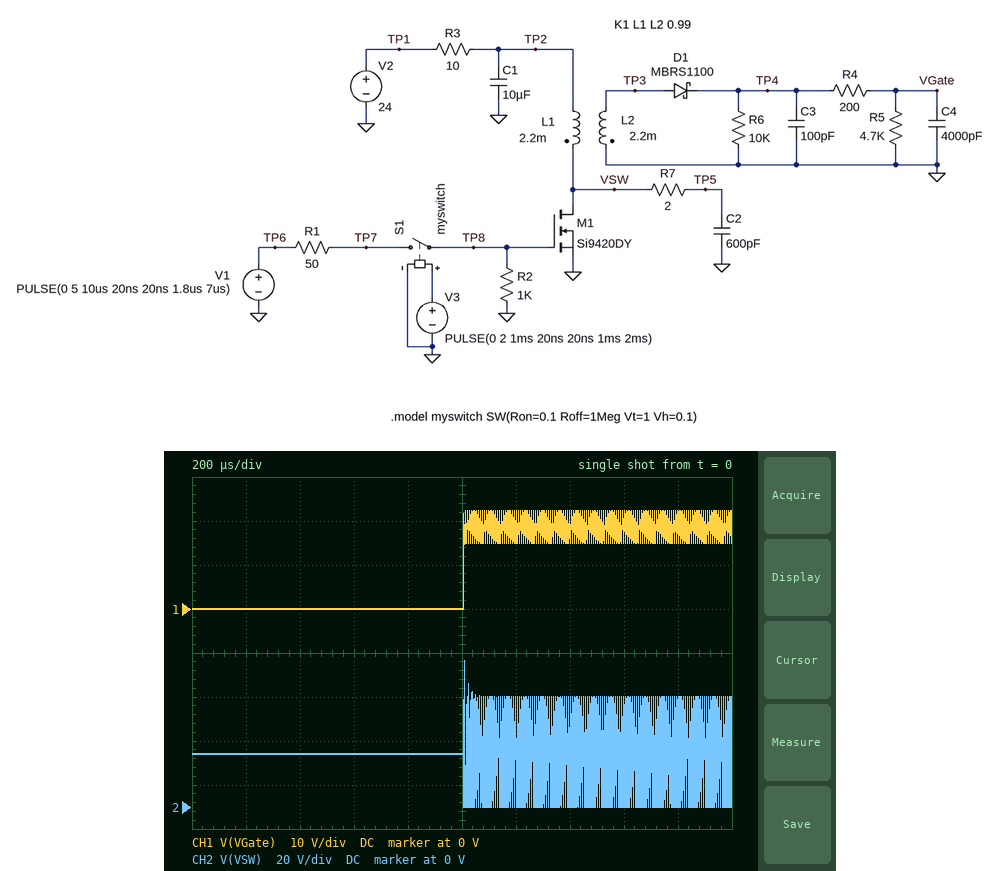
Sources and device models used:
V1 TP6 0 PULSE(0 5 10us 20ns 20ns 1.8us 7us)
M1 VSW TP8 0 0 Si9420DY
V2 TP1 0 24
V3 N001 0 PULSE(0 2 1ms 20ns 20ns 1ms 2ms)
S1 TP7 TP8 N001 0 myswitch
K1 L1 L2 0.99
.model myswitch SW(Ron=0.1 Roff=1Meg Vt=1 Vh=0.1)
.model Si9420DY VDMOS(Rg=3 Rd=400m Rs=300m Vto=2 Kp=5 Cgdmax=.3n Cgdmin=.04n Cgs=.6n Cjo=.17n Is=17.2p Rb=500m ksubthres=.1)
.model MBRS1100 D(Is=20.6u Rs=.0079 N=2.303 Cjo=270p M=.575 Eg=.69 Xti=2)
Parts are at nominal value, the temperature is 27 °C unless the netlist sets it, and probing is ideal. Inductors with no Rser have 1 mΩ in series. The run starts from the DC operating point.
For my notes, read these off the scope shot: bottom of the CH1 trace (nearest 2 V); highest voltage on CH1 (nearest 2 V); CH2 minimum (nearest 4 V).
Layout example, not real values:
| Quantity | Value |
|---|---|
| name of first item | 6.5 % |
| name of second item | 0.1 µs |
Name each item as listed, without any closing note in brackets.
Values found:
| Quantity | Value |
|---|---|
| bottom of the CH1 trace | 0 V |
| highest voltage on CH1 | 22 V |
| CH2 minimum | 0 V |
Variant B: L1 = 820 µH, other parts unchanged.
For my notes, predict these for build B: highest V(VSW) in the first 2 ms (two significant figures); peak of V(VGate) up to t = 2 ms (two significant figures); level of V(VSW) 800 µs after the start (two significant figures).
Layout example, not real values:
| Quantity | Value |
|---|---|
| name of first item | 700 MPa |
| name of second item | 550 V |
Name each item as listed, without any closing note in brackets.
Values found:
| Quantity | Value |
|---|---|
| highest V(VSW) in the first 2 ms | 87 V |
| peak of V(VGate) up to t = 2 ms | 37 V |
| level of V(VSW) 800 µs after the start | 24 V |
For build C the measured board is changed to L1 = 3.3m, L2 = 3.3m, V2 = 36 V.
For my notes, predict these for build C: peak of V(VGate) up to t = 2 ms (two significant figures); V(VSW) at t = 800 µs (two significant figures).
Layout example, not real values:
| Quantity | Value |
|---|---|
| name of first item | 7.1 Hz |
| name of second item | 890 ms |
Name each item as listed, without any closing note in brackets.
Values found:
| Quantity | Value |
|---|---|
| peak of V(VGate) up to t = 2 ms | 34 V |
| V(VSW) at t = 800 µs | 36 V |
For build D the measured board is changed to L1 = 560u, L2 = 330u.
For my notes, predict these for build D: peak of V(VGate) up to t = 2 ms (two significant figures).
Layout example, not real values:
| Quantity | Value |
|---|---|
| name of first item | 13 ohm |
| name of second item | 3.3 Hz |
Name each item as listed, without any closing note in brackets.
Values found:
| Quantity | Value |
|---|---|
| peak of V(VGate) up to t = 2 ms | 17 V |
